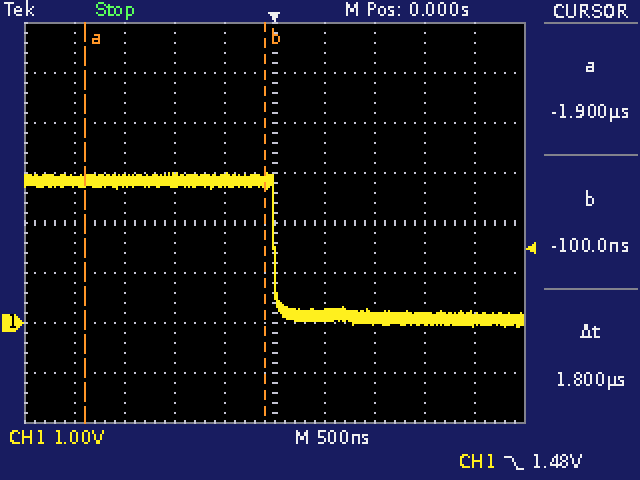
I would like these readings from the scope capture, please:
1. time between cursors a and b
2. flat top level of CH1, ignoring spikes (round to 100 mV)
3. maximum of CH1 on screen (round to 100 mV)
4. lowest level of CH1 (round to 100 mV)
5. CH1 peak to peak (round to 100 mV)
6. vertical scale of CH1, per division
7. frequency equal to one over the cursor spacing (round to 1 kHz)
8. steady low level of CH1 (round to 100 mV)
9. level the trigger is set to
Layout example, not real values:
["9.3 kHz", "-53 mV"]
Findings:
["1.8 µs", "2.8 V", "3.0 V", "-100 mV", "3.1 V", "1 V", "556 kHz", "100 mV", "1.48 V"]
